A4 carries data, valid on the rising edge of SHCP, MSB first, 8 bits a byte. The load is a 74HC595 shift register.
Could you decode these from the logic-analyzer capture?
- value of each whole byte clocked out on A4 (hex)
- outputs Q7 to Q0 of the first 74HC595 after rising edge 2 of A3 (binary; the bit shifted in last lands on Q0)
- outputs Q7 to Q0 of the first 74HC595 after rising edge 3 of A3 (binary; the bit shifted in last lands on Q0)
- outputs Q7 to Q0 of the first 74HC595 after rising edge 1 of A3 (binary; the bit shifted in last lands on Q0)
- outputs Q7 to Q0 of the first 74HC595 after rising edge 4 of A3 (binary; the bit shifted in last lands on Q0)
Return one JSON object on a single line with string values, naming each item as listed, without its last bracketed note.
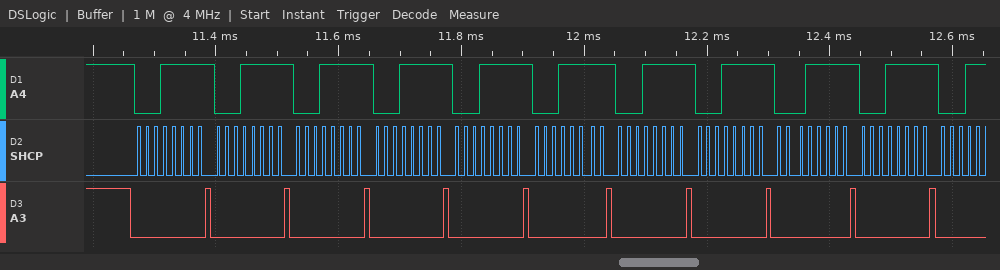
{"value of each whole byte clocked out on A4": "1F 1F 1F 1F 1F 1F 1F 1F 1F 1F", "outputs Q7 to Q0 of the first 74HC595 after rising edge 2 of A3": "00011111", "outputs Q7 to Q0 of the first 74HC595 after rising edge 3 of A3": "00011111", "outputs Q7 to Q0 of the first 74HC595 after rising edge 1 of A3": "00011111", "outputs Q7 to Q0 of the first 74HC595 after rising edge 4 of A3": "00011111"}
